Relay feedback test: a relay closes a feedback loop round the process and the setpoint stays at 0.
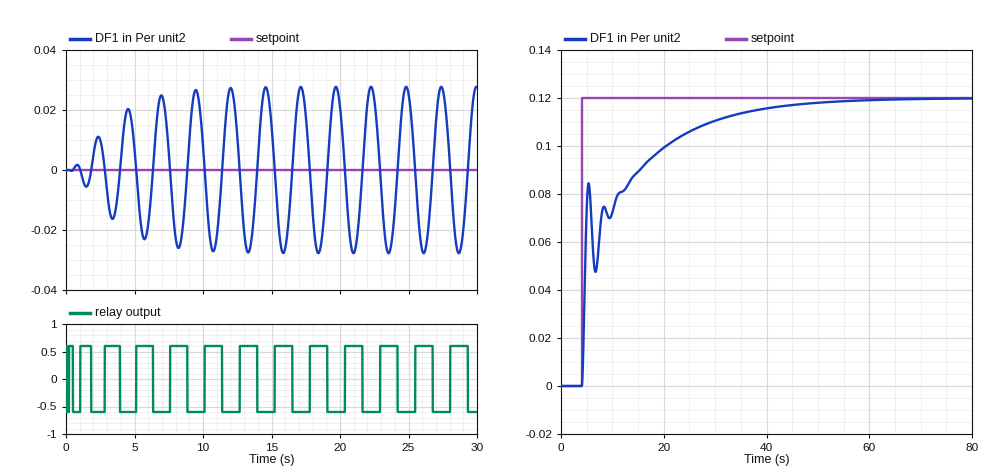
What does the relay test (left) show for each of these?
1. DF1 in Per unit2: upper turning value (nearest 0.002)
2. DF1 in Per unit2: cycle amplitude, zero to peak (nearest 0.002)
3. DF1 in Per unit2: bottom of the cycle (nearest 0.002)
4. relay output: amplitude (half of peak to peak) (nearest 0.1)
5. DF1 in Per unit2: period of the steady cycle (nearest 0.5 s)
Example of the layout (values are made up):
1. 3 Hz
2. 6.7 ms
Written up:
1. 0.028
2. 0.028
3. -0.028
4. 0.6
5. 2.5 s
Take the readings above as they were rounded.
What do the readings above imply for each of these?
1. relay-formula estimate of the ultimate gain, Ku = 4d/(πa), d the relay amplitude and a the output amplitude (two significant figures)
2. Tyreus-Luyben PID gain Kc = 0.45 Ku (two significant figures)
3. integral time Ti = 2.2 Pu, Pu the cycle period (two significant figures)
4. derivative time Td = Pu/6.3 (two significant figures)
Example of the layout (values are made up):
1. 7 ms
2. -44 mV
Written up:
1. 27
2. 12
3. 5.5 s
4. 0.40 s
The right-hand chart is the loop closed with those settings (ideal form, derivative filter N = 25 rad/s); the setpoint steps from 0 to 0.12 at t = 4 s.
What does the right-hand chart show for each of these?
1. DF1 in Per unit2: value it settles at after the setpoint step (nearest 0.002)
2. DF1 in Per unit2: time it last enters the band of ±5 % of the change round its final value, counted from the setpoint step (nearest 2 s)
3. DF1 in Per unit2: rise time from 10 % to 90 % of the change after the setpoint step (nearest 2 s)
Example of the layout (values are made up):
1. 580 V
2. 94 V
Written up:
1. 0.120
2. 32 s
3. 22 s
